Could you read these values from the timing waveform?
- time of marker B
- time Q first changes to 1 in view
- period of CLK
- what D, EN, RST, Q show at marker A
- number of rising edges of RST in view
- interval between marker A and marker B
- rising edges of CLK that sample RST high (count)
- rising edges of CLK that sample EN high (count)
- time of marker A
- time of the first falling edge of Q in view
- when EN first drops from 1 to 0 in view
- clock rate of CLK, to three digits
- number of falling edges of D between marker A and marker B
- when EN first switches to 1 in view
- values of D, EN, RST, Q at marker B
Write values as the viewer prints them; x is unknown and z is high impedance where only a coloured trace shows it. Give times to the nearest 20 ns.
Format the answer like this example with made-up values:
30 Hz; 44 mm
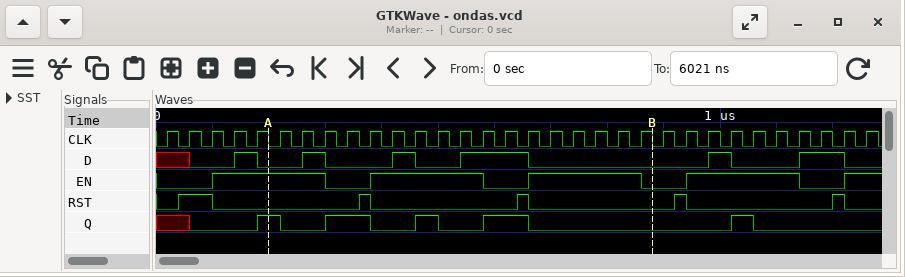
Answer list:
880 ns; 180 ns; 40 ns; D=0, EN=1, RST=0, Q=1; 5; 680 ns; 6; 21; 200 ns; 220 ns; 300 ns; 25.0 MHz; 3; 100 ns; D=0, EN=0, RST=0, Q=0
